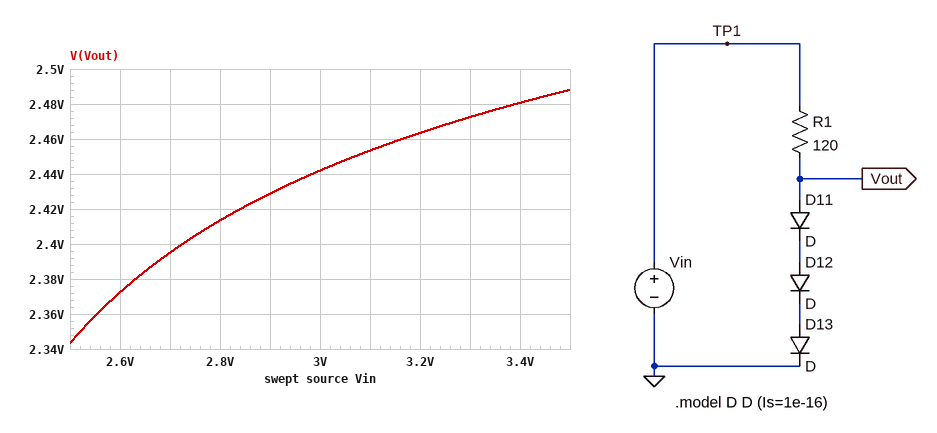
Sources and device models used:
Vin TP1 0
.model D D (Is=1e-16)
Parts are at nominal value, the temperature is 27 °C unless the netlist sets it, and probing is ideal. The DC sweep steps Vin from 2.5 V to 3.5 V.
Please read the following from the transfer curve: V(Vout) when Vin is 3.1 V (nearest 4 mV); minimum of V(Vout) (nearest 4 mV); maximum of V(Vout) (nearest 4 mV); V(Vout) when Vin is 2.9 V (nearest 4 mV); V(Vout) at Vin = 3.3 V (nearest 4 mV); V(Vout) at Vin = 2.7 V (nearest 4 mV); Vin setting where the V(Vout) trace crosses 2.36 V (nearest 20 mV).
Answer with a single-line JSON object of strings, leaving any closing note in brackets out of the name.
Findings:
{"V(Vout) when Vin is 3.1 V": "2.452 V", "minimum of V(Vout)": "2.344 V", "maximum of V(Vout)": "2.488 V", "V(Vout) when Vin is 2.9 V": "2.428 V", "V(Vout) at Vin = 3.3 V": "2.472 V", "V(Vout) at Vin = 2.7 V": "2.396 V", "Vin setting where the V(Vout) trace crosses 2.36 V": "2.56 V"}
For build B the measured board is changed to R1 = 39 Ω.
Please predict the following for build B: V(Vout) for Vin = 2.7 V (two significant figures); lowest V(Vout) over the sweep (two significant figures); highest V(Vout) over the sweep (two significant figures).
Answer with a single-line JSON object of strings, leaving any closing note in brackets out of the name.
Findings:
{"V(Vout) for Vin = 2.7 V": "2.5 V", "lowest V(Vout) over the sweep": "2.4 V", "highest V(Vout) over the sweep": "2.6 V"}
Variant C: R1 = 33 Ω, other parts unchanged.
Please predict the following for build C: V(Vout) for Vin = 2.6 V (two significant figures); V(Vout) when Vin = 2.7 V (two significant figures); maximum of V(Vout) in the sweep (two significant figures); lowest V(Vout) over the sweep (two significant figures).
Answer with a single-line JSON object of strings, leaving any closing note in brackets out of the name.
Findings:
{"V(Vout) for Vin = 2.6 V": "2.4 V", "V(Vout) when Vin = 2.7 V": "2.5 V", "maximum of V(Vout) in the sweep": "2.6 V", "lowest V(Vout) over the sweep": "2.4 V"}
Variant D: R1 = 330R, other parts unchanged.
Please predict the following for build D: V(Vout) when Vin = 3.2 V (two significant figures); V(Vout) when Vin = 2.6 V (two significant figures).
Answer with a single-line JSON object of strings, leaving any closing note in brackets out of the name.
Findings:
{"V(Vout) when Vin = 3.2 V": "2.4 V", "V(Vout) when Vin = 2.6 V": "2.3 V"}
